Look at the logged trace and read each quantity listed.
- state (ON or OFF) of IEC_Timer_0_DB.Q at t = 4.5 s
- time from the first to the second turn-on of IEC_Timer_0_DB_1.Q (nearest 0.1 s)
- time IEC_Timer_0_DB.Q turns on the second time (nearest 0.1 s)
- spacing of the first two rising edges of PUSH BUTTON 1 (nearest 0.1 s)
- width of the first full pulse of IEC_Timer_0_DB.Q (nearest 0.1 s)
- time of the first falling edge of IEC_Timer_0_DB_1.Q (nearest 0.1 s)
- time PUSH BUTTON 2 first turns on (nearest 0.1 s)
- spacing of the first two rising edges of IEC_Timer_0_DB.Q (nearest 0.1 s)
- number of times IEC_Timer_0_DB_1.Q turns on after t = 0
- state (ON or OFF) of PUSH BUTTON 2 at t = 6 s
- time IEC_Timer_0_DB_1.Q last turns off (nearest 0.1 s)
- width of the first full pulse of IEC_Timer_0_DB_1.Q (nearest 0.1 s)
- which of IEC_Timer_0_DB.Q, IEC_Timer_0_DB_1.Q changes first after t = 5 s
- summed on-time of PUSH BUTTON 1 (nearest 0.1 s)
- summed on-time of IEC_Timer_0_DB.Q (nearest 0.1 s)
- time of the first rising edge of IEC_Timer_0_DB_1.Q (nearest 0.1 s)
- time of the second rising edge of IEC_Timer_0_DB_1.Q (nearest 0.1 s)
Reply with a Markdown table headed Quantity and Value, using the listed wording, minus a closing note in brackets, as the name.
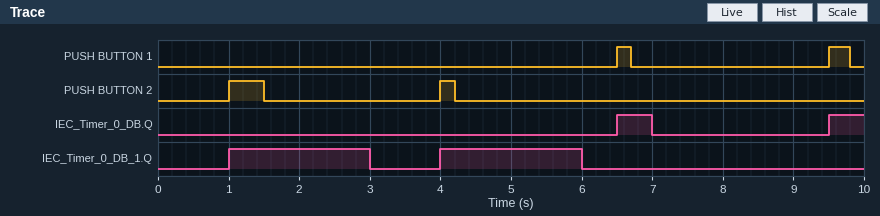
| Quantity | Value |
|---|---|
| state (ON or OFF) of IEC_Timer_0_DB.Q at t = 4.5 s | OFF |
| time from the first to the second turn-on of IEC_Timer_0_DB_1.Q | 3.0 s |
| time IEC_Timer_0_DB.Q turns on the second time | 9.5 s |
| spacing of the first two rising edges of PUSH BUTTON 1 | 3.0 s |
| width of the first full pulse of IEC_Timer_0_DB.Q | 0.5 s |
| time of the first falling edge of IEC_Timer_0_DB_1.Q | 3.0 s |
| time PUSH BUTTON 2 first turns on | 1.0 s |
| spacing of the first two rising edges of IEC_Timer_0_DB.Q | 3.0 s |
| number of times IEC_Timer_0_DB_1.Q turns on after t = 0 | 2 |
| state (ON or OFF) of PUSH BUTTON 2 at t = 6 s | OFF |
| time IEC_Timer_0_DB_1.Q last turns off | 6.0 s |
| width of the first full pulse of IEC_Timer_0_DB_1.Q | 2.0 s |
| which of IEC_Timer_0_DB.Q, IEC_Timer_0_DB_1.Q changes first after t = 5 s | IEC_Timer_0_DB_1.Q |
| summed on-time of PUSH BUTTON 1 | 0.5 s |
| summed on-time of IEC_Timer_0_DB.Q | 1.0 s |
| time of the first rising edge of IEC_Timer_0_DB_1.Q | 1.0 s |
| time of the second rising edge of IEC_Timer_0_DB_1.Q | 4.0 s |
